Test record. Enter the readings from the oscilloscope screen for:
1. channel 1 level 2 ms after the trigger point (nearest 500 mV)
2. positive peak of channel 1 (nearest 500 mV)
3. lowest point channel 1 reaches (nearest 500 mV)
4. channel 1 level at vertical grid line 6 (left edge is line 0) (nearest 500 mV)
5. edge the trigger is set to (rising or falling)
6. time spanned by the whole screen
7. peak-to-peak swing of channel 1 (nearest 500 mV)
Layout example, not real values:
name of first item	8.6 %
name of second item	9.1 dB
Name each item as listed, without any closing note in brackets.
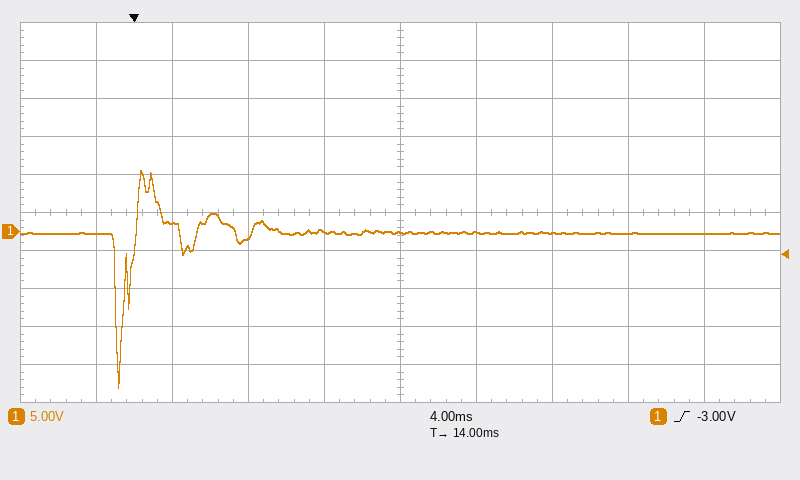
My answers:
channel 1 level 2 ms after the trigger point	1.0 V
positive peak of channel 1	8.0 V
lowest point channel 1 reaches	-20.5 V
channel 1 level at vertical grid line 6 (left edge is line 0)	0.0 V
edge the trigger is set to	rising
time spanned by the whole screen	40 ms
peak-to-peak swing of channel 1	28.5 V
